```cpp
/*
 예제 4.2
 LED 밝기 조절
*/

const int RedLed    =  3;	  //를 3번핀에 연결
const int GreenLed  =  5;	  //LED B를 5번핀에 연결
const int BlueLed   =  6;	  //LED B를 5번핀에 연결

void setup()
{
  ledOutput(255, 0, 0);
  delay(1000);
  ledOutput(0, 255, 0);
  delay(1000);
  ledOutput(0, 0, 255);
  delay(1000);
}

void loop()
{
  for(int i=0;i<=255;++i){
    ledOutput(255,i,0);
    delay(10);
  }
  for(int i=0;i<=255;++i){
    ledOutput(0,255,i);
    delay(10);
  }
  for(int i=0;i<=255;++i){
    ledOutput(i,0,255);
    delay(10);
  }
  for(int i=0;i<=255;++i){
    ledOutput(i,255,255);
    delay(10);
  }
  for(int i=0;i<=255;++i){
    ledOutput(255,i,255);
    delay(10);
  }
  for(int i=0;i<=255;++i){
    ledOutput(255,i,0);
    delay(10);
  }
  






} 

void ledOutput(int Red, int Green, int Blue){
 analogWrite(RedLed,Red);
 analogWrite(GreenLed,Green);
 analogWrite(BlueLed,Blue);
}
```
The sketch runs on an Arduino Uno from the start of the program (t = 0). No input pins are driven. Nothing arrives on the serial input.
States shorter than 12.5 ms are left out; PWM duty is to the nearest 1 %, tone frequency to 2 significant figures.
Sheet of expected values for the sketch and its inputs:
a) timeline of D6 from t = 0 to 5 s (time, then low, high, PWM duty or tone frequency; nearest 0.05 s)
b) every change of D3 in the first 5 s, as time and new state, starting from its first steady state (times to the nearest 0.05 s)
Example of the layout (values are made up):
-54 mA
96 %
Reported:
0 s low; 2 s high; 3 s low
0 s high; 1 s low; 3 s high
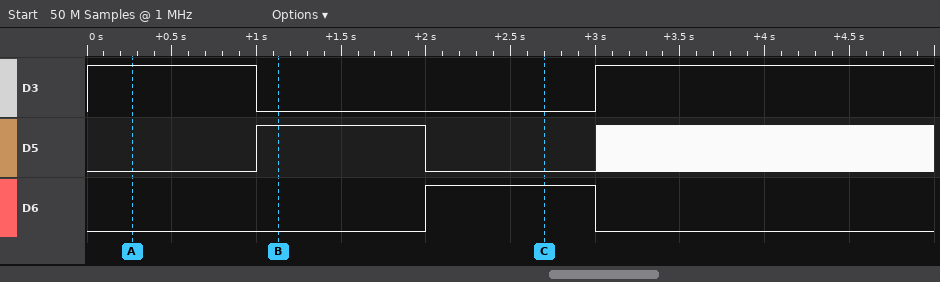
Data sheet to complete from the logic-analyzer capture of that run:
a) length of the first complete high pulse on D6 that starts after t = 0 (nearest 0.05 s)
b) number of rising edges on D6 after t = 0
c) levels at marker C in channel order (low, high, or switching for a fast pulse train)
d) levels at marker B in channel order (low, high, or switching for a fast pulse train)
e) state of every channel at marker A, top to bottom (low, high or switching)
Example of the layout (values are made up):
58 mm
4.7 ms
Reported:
1.00 s
1
D3 low, D5 low, D6 high
D3 low, D5 high, D6 low
D3 high, D5 low, D6 low
